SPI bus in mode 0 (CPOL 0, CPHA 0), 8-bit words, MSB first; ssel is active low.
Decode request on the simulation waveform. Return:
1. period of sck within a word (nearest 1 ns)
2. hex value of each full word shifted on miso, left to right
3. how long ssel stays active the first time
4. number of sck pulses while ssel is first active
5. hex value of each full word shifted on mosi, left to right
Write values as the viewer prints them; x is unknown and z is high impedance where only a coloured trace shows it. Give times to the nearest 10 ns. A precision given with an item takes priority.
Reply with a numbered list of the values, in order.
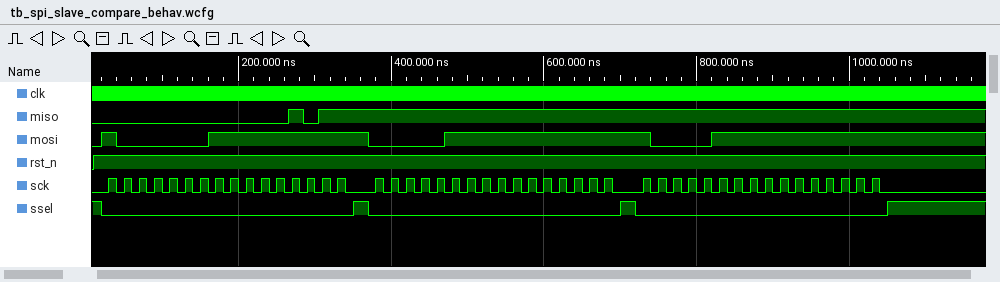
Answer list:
1. 20 ns
2. 00, 0B, FF, FF, FF, FF
3. 330 ns
4. 16
5. 81, FF, 07, FF, 87, FF
